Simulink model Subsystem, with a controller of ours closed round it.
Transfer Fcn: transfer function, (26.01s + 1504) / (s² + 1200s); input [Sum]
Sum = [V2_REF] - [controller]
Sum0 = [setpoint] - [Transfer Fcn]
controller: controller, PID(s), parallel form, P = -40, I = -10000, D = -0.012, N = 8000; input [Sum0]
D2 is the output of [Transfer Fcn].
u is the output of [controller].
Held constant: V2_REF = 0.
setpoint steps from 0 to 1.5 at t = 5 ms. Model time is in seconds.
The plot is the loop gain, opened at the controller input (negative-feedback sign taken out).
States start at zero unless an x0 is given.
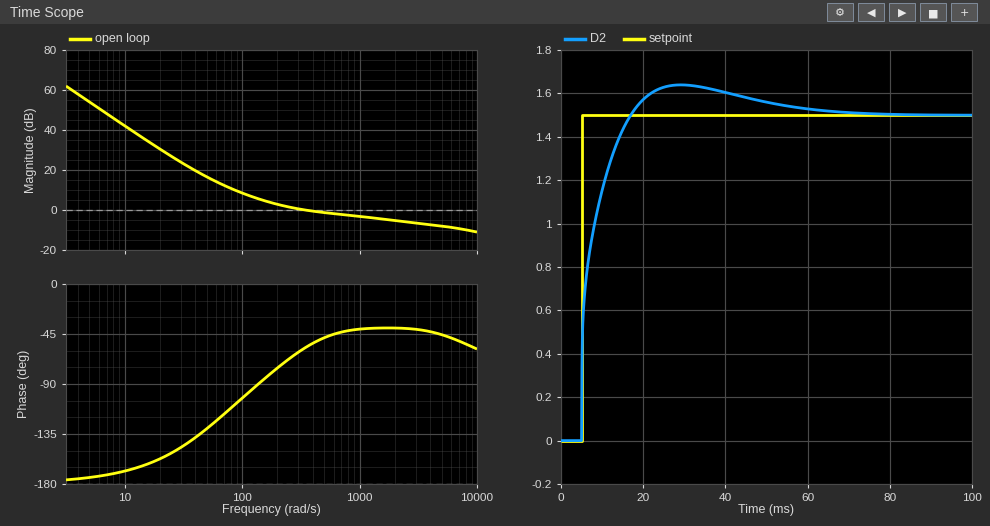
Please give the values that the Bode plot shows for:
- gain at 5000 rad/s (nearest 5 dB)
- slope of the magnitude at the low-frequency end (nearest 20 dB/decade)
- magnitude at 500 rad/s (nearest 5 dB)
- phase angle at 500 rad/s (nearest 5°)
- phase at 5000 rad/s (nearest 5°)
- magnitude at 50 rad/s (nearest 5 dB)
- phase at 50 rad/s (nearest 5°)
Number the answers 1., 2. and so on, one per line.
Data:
1. -10 dB
2. -40 dB/decade
3. 0 dB
4. -50°
5. -45°
6. 15 dB
7. -130°
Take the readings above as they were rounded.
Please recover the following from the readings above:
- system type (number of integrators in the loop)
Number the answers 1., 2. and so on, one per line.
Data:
1. 2
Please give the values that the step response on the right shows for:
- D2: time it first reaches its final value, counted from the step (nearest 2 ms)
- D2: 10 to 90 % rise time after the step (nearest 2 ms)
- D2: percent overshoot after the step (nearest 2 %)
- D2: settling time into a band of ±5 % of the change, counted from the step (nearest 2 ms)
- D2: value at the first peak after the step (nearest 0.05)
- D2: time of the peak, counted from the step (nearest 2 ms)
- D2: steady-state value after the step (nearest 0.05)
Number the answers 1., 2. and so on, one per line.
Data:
1. 12 ms
2. 8 ms
3. 10 %
4. 42 ms
5. 1.65
6. 24 ms
7. 1.50
